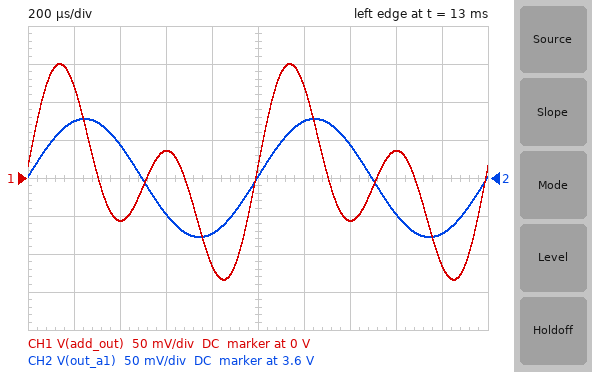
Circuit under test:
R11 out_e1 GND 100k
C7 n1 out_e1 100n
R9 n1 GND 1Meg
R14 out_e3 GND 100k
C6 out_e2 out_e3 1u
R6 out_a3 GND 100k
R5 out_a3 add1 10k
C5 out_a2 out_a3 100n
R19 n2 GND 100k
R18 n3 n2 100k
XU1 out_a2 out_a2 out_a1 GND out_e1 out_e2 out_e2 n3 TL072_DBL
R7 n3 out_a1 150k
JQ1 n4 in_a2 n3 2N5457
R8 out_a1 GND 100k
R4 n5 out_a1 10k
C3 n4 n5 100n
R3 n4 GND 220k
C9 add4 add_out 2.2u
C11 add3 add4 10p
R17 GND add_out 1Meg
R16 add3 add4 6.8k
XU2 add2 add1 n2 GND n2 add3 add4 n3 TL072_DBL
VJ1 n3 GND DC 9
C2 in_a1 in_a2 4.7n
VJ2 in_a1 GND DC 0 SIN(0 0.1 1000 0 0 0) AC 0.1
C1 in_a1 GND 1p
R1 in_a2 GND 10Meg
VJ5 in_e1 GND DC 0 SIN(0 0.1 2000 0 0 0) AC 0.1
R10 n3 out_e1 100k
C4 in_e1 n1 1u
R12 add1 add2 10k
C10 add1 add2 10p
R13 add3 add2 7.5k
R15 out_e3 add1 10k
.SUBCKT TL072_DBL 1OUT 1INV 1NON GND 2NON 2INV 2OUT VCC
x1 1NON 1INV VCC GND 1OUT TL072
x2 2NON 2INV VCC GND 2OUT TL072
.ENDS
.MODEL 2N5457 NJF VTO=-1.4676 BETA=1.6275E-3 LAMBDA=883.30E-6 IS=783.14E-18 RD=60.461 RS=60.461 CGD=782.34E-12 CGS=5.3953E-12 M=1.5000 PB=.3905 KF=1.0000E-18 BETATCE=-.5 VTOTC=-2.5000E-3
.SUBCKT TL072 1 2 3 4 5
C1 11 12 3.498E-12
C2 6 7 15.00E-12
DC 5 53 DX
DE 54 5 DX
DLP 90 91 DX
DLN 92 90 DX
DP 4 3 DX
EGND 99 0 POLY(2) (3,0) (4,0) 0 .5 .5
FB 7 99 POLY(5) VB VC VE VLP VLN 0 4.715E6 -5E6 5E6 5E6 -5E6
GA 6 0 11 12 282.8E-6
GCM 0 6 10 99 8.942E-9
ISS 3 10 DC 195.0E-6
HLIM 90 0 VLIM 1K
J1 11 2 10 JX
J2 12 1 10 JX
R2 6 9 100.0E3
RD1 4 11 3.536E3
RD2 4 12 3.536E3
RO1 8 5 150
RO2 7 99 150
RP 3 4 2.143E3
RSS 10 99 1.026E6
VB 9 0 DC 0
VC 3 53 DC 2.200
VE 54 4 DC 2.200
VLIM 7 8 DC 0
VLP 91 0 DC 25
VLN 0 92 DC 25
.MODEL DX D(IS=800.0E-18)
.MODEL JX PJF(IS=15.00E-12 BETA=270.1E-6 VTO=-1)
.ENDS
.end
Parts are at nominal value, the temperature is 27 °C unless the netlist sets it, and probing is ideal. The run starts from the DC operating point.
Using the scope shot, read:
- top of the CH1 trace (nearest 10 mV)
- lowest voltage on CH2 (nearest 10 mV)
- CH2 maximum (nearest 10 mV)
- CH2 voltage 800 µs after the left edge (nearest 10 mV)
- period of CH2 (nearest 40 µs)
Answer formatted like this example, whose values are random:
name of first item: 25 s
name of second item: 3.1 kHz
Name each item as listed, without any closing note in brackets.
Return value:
top of the CH1 trace: 150 mV
lowest voltage on CH2: 3.52 V
CH2 maximum: 3.68 V
CH2 voltage 800 µs after the left edge: 3.53 V
period of CH2: 1.00 ms
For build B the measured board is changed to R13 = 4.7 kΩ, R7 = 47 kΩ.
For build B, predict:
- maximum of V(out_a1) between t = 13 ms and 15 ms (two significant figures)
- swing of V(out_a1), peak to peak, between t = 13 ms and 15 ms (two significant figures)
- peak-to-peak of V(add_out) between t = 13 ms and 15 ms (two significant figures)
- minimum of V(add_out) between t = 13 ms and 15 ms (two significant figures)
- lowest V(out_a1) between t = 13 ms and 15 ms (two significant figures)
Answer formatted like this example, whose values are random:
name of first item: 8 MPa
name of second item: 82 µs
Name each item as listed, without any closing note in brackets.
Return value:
maximum of V(out_a1) between t = 13 ms and 15 ms: 6.2 V
swing of V(out_a1), peak to peak, between t = 13 ms and 15 ms: 130 mV
peak-to-peak of V(add_out) between t = 13 ms and 15 ms: 430 mV
minimum of V(add_out) between t = 13 ms and 15 ms: -200 mV
lowest V(out_a1) between t = 13 ms and 15 ms: 6.1 V
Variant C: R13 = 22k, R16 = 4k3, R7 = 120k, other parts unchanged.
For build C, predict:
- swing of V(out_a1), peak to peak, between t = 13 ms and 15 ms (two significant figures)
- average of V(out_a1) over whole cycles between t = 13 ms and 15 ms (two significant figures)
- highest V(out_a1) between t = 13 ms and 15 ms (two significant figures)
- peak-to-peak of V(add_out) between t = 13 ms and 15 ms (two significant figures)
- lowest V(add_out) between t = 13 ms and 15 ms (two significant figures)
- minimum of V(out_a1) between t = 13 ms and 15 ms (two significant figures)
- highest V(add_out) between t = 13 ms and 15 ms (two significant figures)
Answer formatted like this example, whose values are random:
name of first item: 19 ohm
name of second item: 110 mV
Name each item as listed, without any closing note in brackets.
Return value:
swing of V(out_a1), peak to peak, between t = 13 ms and 15 ms: 150 mV
average of V(out_a1) over whole cycles between t = 13 ms and 15 ms: 4.1 V
highest V(out_a1) between t = 13 ms and 15 ms: 4.2 V
peak-to-peak of V(add_out) between t = 13 ms and 15 ms: 61 mV
lowest V(add_out) between t = 13 ms and 15 ms: -29 mV
minimum of V(out_a1) between t = 13 ms and 15 ms: 4.0 V
highest V(add_out) between t = 13 ms and 15 ms: 32 mV
